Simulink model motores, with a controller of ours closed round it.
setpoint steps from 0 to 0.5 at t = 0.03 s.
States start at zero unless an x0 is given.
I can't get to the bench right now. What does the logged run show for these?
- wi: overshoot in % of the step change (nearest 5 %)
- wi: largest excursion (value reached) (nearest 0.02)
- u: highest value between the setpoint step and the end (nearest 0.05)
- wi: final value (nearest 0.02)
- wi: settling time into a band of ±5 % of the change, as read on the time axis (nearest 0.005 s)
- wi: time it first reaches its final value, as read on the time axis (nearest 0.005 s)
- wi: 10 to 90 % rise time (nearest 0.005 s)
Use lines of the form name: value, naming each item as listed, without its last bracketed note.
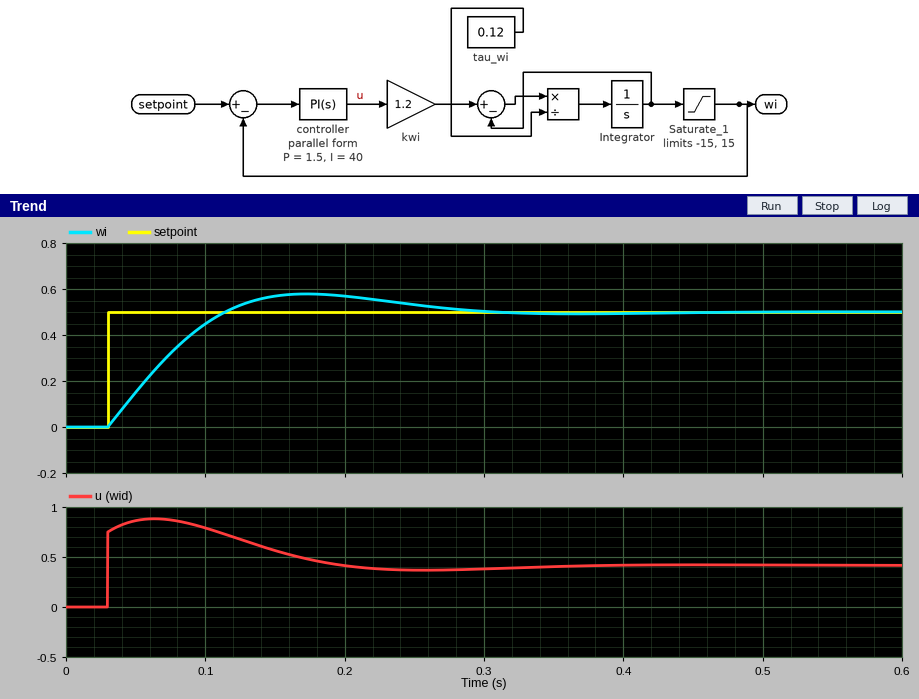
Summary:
wi: overshoot in % of the step change: 15 %
wi: largest excursion (value reached): 0.58
u: highest value between the setpoint step and the end: 0.90
wi: final value: 0.50
wi: settling time into a band of ±5 % of the change, as read on the time axis: 0.260 s
wi: time it first reaches its final value, as read on the time axis: 0.115 s
wi: 10 to 90 % rise time: 0.065 s
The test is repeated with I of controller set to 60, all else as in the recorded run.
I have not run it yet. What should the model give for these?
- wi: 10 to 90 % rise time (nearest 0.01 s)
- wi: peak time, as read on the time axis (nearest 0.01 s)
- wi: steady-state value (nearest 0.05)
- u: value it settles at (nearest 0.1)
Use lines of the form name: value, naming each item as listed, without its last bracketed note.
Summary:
wi: 10 to 90 % rise time: 0.05 s
wi: peak time, as read on the time axis: 0.15 s
wi: steady-state value: 0.50
u: value it settles at: 0.4
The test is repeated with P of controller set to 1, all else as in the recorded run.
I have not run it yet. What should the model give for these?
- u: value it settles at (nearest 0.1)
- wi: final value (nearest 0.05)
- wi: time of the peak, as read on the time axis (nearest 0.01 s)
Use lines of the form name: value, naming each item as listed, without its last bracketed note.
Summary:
u: value it settles at: 0.4
wi: final value: 0.50
wi: time of the peak, as read on the time axis: 0.18 s
